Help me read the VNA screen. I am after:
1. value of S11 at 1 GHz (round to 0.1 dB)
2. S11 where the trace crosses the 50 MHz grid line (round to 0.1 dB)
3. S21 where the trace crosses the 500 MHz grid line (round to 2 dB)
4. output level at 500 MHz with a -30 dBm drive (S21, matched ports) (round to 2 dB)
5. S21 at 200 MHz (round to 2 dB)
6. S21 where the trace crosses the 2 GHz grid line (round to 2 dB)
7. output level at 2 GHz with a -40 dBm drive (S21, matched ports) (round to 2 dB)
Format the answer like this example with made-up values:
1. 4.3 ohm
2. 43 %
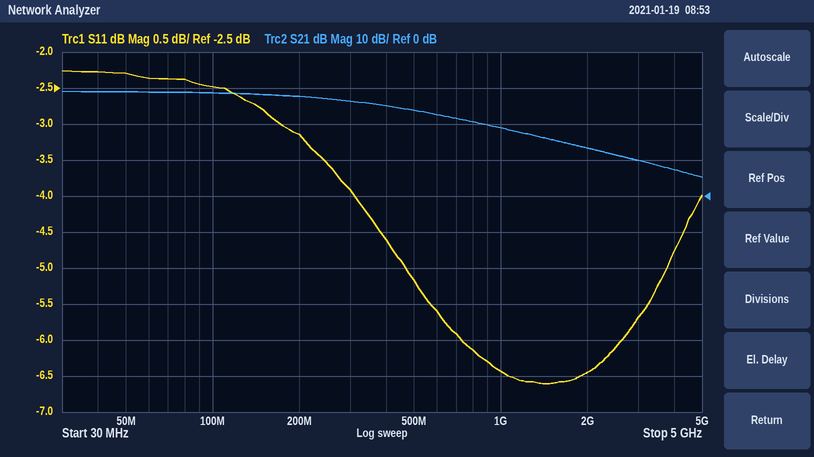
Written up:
1. -6.4 dB
2. -2.3 dB
3. 24 dB
4. -6 dBm
5. 28 dB
6. 14 dB
7. -26 dBm
